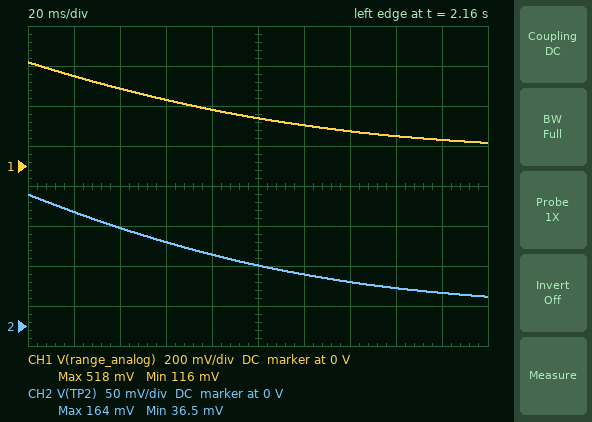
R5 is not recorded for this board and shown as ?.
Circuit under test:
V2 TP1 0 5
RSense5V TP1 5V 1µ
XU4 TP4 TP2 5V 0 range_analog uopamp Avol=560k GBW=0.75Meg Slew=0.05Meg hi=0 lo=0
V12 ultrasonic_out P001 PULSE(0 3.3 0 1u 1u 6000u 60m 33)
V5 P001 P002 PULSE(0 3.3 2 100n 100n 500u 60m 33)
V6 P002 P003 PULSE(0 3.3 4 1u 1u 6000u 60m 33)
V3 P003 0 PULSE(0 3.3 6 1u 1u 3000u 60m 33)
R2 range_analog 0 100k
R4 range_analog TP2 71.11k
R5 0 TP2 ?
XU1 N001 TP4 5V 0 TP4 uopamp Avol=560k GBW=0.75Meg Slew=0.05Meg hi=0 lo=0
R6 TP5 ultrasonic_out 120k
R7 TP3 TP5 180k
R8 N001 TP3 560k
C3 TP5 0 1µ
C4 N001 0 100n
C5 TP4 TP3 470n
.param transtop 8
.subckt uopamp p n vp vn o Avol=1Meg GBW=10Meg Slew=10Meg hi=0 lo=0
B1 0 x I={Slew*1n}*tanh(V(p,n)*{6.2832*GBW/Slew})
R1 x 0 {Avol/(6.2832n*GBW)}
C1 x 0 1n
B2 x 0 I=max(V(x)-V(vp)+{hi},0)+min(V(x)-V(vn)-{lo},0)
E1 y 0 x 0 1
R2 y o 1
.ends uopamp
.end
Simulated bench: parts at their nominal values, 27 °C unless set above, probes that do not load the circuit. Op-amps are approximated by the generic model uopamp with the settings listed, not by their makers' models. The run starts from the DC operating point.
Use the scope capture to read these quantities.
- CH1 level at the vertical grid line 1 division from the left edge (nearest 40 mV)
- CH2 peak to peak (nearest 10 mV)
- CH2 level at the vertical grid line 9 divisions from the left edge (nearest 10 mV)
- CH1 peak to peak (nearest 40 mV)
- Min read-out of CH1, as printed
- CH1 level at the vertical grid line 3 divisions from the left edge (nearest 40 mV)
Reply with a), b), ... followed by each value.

a) 440 mV
b) 130 mV
c) 40 mV
d) 400 mV
e) 116 mV
f) 320 mV
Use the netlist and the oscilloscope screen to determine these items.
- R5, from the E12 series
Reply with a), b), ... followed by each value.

a) 33 kΩ
